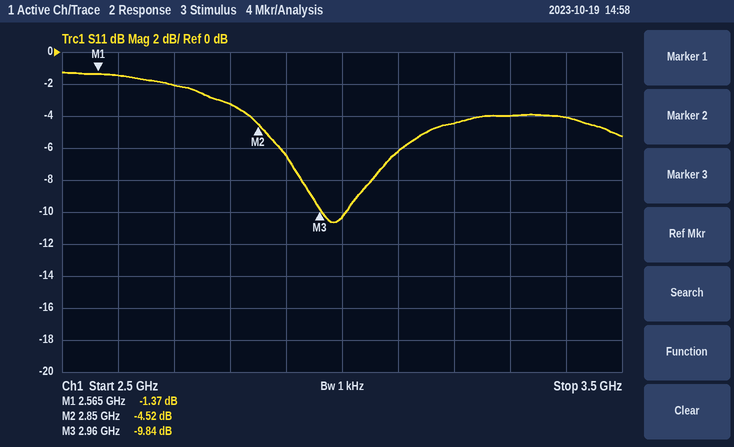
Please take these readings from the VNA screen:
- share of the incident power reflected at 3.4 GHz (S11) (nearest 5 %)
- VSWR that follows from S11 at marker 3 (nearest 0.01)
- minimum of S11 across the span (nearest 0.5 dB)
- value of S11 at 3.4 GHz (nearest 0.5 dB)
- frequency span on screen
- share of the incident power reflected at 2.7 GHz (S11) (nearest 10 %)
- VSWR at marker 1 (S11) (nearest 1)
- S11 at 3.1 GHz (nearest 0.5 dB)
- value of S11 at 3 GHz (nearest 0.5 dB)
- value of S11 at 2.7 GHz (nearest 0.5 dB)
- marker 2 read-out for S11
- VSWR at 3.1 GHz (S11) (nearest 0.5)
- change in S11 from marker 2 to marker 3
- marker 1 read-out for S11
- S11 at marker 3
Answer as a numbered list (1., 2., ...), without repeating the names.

1. 40 %
2. 1.95
3. -10.5 dB
4. -4.0 dB
5. 1 GHz
6. 60 %
7. 13
8. -6.0 dB
9. -10.5 dB
10. -2.0 dB
11. -4.52 dB
12. 3.0
13. -5.32 dB
14. -1.37 dB
15. -9.84 dB
